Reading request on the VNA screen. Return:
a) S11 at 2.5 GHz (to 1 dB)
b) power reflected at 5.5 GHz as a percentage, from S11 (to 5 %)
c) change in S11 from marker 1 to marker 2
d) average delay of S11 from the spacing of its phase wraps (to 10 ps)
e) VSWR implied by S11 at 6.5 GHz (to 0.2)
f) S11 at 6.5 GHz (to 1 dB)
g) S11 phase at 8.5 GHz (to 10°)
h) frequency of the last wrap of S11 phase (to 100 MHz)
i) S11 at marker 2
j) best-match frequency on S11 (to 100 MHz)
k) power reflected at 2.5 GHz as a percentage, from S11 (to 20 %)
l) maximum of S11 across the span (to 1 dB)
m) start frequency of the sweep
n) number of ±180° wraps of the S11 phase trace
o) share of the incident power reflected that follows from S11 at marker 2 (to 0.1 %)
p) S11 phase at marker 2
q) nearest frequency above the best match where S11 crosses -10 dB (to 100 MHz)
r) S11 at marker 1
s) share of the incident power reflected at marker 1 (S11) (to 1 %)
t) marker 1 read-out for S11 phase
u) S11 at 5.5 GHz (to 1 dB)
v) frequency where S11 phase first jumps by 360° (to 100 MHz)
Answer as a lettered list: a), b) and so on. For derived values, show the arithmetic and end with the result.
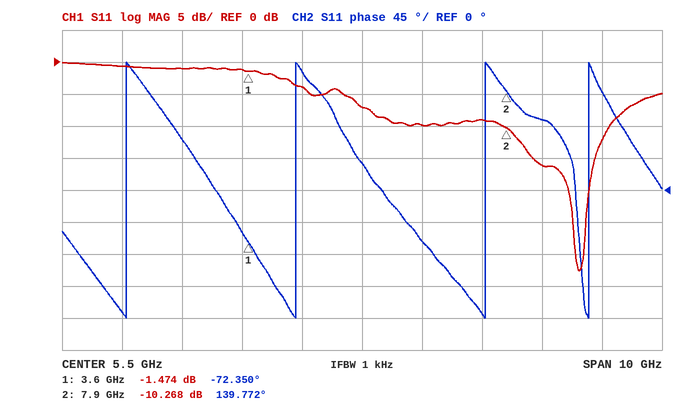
a) -1 dB
b) 10^(-7/10) ≈ 20 %
c) -10.268 − (-1.474) = -8.794 dB
d) 3 cycles / (9.3 GHz − 1.6 GHz) ≈ 390 ps
e) |Γ| = 10^(-10/20) = 0.3162; VSWR = (1 + 0.3162)/(1 − 0.3162) ≈ 1.92, so 2.0 to the nearest 0.2
f) -10 dB
g) 100°
h) 9.3 GHz
i) -10.268 dB
j) 9.1 GHz
k) 10^(-1/10) ≈ 79.4 %, so 80 % to the nearest 20 %
l) 0 dB
m) 500 MHz
n) 4
o) 10^(-10.268/10) ≈ 9.4 %
p) 139.772°
q) 9.6 GHz
r) -1.474 dB
s) 10^(-1.474/10) ≈ 71 %
t) -72.350°
u) -7 dB
v) 1.6 GHz
